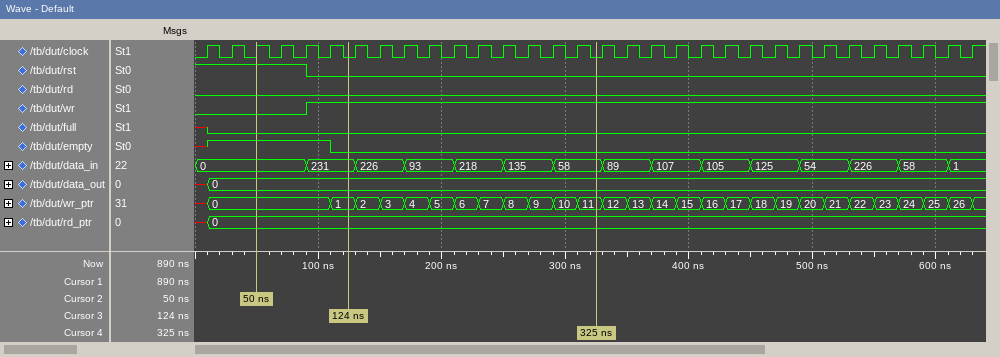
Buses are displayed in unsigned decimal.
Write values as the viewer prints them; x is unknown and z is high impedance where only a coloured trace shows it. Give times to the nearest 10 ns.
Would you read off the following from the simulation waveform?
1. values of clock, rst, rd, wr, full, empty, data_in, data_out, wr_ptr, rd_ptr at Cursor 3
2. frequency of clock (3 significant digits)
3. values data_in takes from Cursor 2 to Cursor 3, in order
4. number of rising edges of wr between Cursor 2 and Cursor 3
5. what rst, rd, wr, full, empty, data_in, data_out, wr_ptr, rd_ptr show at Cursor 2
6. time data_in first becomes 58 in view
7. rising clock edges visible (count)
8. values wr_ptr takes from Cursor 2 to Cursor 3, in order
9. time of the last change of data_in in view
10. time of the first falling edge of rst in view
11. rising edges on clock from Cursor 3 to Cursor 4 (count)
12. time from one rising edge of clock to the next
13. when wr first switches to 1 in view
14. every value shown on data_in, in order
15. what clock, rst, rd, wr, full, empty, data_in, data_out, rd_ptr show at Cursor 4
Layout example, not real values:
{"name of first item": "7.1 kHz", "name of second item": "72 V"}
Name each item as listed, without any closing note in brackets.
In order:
{"values of clock, rst, rd, wr, full, empty, data_in, data_out, wr_ptr, rd_ptr at Cursor 3": "clock=0, rst=0, rd=0, wr=1, full=0, empty=0, data_in=231, data_out=0, wr_ptr=1, rd_ptr=0", "frequency of clock": "50.0 MHz", "values data_in takes from Cursor 2 to Cursor 3, in order": "0, 231", "number of rising edges of wr between Cursor 2 and Cursor 3": "1", "what rst, rd, wr, full, empty, data_in, data_out, wr_ptr, rd_ptr show at Cursor 2": "rst=1, rd=0, wr=0, full=0, empty=1, data_in=0, data_out=0, wr_ptr=0, rd_ptr=0", "time data_in first becomes 58 in view": "290 ns", "rising clock edges visible": "32", "values wr_ptr takes from Cursor 2 to Cursor 3, in order": "0, 1", "time of the last change of data_in in view": "610 ns", "time of the first falling edge of rst in view": "90 ns", "rising edges on clock from Cursor 3 to Cursor 4": "10", "time from one rising edge of clock to the next": "20 ns", "when wr first switches to 1 in view": "90 ns", "every value shown on data_in, in order": "0, 231, 226, 93, 218, 135, 58, 89, 107, 105, 125, 54, 226, 58, 1", "what clock, rst, rd, wr, full, empty, data_in, data_out, rd_ptr show at Cursor 4": "clock=0, rst=0, rd=0, wr=1, full=0, empty=0, data_in=58, data_out=0, rd_ptr=0"}
